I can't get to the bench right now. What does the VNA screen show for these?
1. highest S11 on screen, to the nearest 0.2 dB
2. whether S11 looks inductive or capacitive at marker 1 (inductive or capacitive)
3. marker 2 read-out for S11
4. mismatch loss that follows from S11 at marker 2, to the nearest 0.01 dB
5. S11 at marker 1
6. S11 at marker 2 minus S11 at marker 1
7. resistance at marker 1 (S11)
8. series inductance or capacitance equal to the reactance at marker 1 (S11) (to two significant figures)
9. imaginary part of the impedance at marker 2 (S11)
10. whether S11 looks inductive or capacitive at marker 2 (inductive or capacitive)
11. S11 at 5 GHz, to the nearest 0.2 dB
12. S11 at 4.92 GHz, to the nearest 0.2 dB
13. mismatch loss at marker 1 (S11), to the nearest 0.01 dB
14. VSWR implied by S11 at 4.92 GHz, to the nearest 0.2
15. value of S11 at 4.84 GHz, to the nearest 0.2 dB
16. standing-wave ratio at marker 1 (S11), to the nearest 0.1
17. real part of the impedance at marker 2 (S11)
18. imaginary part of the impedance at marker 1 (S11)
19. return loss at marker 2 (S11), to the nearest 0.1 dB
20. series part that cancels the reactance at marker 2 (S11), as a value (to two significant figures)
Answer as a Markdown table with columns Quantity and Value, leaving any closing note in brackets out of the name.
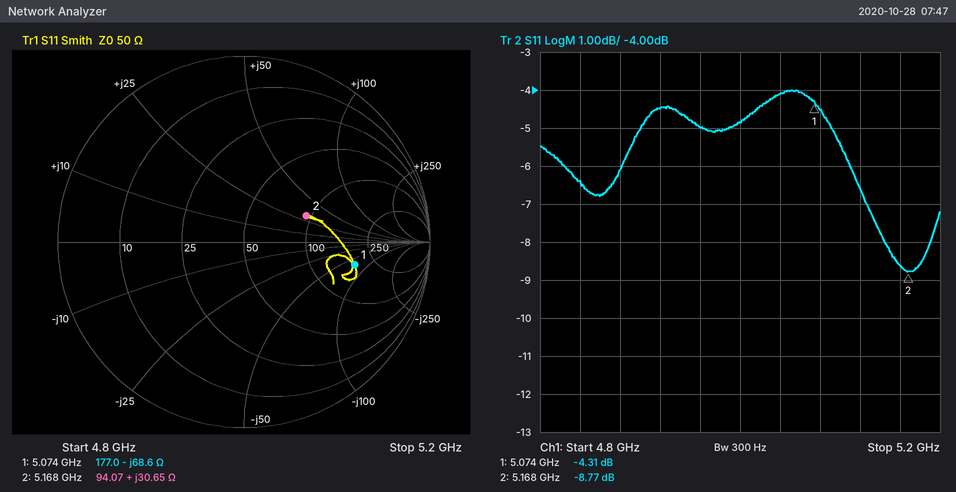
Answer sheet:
| Quantity | Value |
|---|---|
| highest S11 on screen, to the nearest 0.2 dB | -4.0 dB |
| whether S11 looks inductive or capacitive at marker 1 | capacitive |
| marker 2 read-out for S11 | -8.77 dB |
| mismatch loss that follows from S11 at marker 2, to the nearest 0.01 dB | 0.62 dB |
| S11 at marker 1 | -4.31 dB |
| S11 at marker 2 minus S11 at marker 1 | -4.46 dB |
| resistance at marker 1 | 177.0 Ω |
| series inductance or capacitance equal to the reactance at marker 1 (S11) | 460 fF |
| imaginary part of the impedance at marker 2 | +30.65 Ω |
| whether S11 looks inductive or capacitive at marker 2 | inductive |
| S11 at 5 GHz, to the nearest 0.2 dB | -4.8 dB |
| S11 at 4.92 GHz, to the nearest 0.2 dB | -4.4 dB |
| mismatch loss at marker 1 (S11), to the nearest 0.01 dB | 2.01 dB |
| VSWR implied by S11 at 4.92 GHz, to the nearest 0.2 | 4.0 |
| value of S11 at 4.84 GHz, to the nearest 0.2 dB | -6.4 dB |
| standing-wave ratio at marker 1 (S11), to the nearest 0.1 | 4.1 |
| real part of the impedance at marker 2 | 94.07 Ω |
| imaginary part of the impedance at marker 1 | -68.6 Ω |
| return loss at marker 2 (S11), to the nearest 0.1 dB | 8.8 dB |
| series part that cancels the reactance at marker 2 (S11), as a value | 1.0 pF |
